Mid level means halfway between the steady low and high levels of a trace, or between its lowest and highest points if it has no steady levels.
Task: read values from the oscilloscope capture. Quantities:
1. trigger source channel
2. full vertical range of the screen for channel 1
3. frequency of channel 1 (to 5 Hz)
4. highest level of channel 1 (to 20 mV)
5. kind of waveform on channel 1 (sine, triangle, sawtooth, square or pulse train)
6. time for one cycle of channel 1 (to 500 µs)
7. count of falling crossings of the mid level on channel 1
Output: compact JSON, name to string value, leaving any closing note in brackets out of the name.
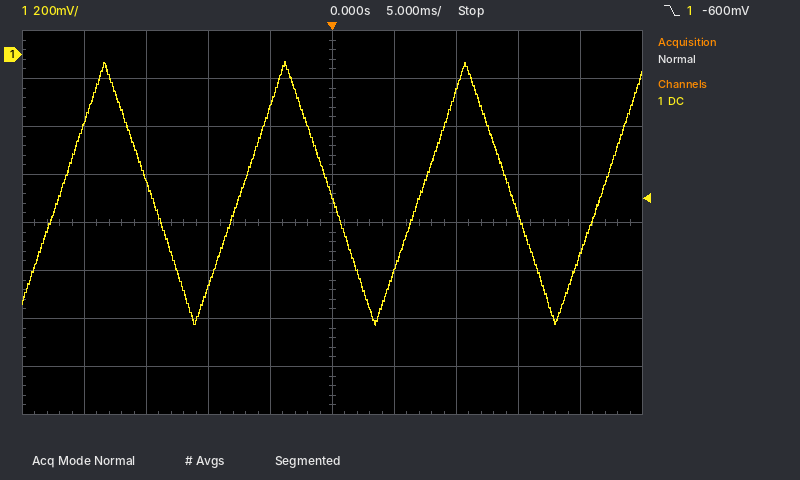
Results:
{"trigger source channel": "channel 1", "full vertical range of the screen for channel 1": "1.6 V", "frequency of channel 1": "70 Hz", "highest level of channel 1": "-20 mV", "kind of waveform on channel 1": "triangle", "time for one cycle of channel 1": "14.5 ms", "count of falling crossings of the mid level on channel 1": "3"}
